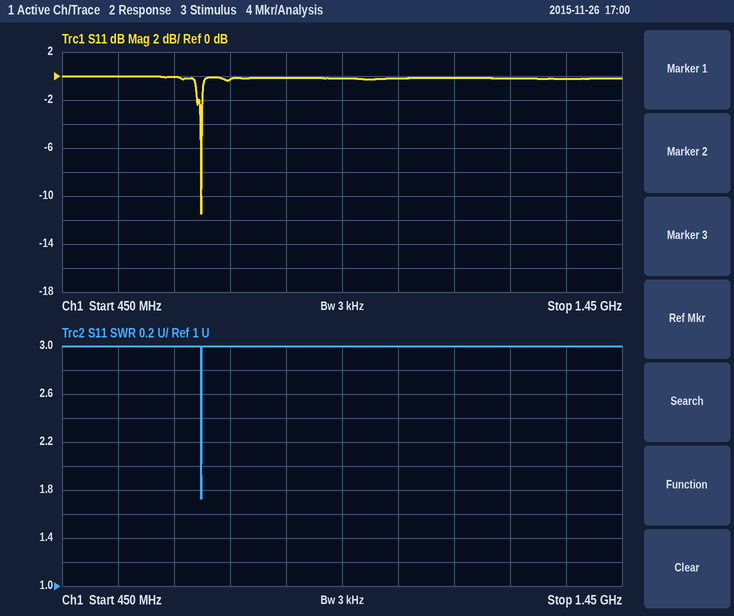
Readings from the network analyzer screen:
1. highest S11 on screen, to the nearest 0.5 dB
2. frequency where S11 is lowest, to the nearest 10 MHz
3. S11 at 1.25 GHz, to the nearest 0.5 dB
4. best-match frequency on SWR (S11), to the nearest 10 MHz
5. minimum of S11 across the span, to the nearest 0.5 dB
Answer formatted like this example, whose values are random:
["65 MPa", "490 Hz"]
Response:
["0.0 dB", "700 MHz", "0.0 dB", "700 MHz", "-11.5 dB"]
